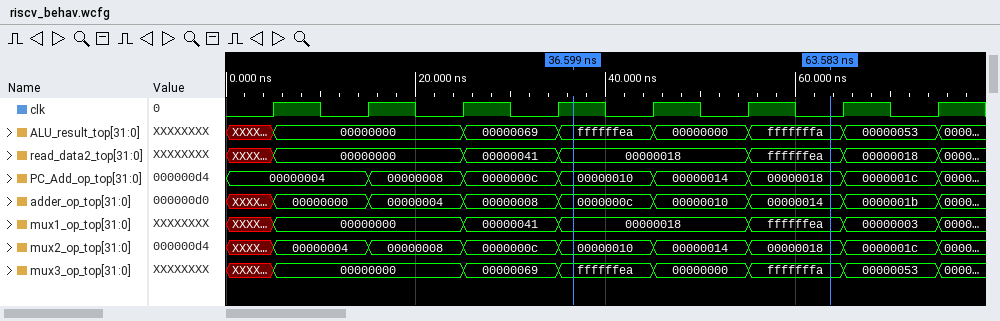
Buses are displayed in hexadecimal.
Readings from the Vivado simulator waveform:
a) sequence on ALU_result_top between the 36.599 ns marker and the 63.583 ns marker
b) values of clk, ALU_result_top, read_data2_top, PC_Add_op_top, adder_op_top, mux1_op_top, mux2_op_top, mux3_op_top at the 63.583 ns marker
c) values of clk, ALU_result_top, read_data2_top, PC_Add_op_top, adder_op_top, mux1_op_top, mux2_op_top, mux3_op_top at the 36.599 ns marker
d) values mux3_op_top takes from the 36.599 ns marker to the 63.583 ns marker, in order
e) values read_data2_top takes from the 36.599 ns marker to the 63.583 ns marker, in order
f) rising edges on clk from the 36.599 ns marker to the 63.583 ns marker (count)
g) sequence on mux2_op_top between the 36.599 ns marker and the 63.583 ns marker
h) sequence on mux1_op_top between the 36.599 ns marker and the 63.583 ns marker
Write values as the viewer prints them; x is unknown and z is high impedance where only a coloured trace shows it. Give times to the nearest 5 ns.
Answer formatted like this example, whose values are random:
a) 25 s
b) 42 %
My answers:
a) ffffffea, 00000000, fffffffa
b) clk=0, ALU_result_top=fffffffa, read_data2_top=ffffffea, PC_Add_op_top=00000018, adder_op_top=00000014, mux1_op_top=ffffffea, mux2_op_top=00000018, mux3_op_top=fffffffa
c) clk=1, ALU_result_top=ffffffea, read_data2_top=00000018, PC_Add_op_top=00000010, adder_op_top=0000000c, mux1_op_top=00000018, mux2_op_top=00000010, mux3_op_top=ffffffea
d) ffffffea, 00000000, fffffffa
e) 00000018, ffffffea
f) 2
g) 00000010, 00000014, 00000018
h) 00000018, ffffffea
